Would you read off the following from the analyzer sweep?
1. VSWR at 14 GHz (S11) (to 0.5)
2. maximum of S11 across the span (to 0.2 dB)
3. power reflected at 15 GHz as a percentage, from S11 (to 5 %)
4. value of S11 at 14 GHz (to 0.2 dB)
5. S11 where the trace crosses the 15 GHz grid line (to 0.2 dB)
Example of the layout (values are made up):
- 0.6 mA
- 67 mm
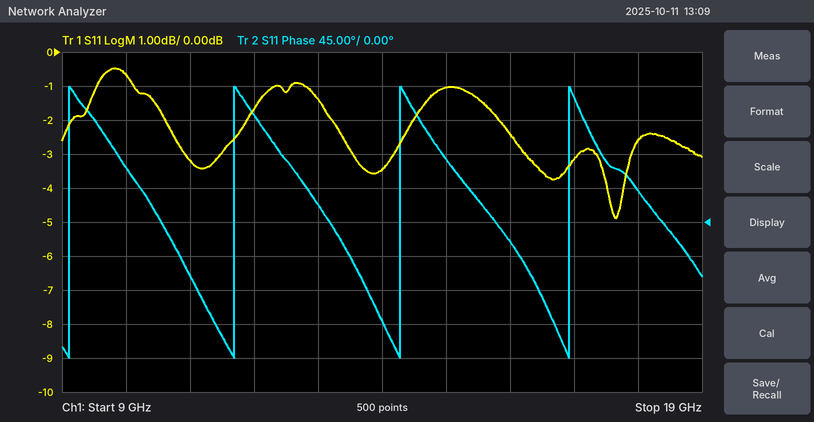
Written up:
- 5.0
- -0.4 dB
- 80 %
- -3.4 dB
- -1.0 dB
